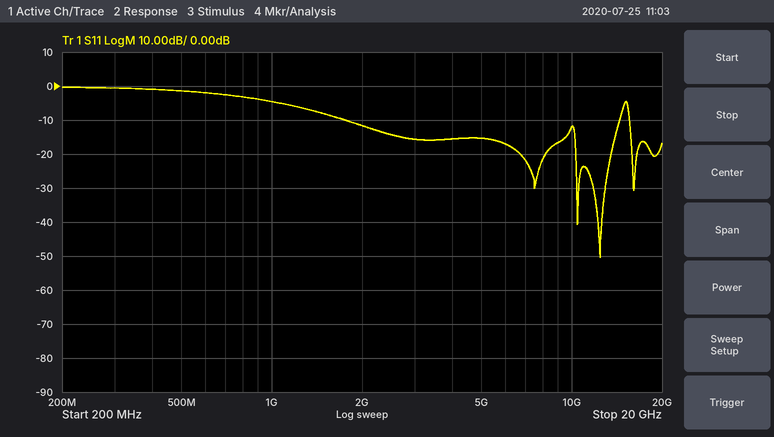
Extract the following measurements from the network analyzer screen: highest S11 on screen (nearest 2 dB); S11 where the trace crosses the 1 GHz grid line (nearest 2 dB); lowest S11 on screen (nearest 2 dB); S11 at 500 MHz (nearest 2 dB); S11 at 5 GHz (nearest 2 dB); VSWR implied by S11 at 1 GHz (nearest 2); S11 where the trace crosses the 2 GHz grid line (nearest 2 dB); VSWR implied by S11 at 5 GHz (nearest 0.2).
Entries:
0 dB
-4 dB
-50 dB
-2 dB
-16 dB
4
-12 dB
1.4
